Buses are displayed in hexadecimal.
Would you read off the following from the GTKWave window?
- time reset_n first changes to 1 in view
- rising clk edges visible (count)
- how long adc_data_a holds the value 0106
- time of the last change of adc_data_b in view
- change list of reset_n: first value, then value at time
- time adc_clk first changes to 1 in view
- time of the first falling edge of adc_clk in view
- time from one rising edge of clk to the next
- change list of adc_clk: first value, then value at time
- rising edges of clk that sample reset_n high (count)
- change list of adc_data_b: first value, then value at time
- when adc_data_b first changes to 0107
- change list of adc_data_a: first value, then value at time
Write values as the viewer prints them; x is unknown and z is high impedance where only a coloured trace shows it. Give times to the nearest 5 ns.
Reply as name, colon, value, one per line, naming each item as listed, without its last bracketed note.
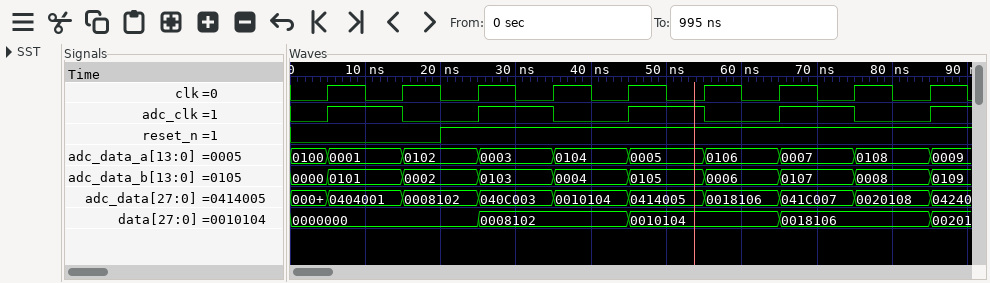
time reset_n first changes to 1 in view: 20 ns
rising clk edges visible: 9
how long adc_data_a holds the value 0106: 10 ns
time of the last change of adc_data_b in view: 85 ns
change list of reset_n: first value, then value at time: 0, 1 at 20 ns
time adc_clk first changes to 1 in view: 5 ns
time of the first falling edge of adc_clk in view: 15 ns
time from one rising edge of clk to the next: 10 ns
change list of adc_clk: first value, then value at time: 0, 1 at 5 ns, 0 at 15 ns, 1 at 25 ns, 0 at 35 ns, 1 at 45 ns, 0 at 55 ns, 1 at 65 ns, 0 at 75 ns, 1 at 85 ns
rising edges of clk that sample reset_n high: 7
change list of adc_data_b: first value, then value at time: 0000, 0101 at 5 ns, 0002 at 15 ns, 0103 at 25 ns, 0004 at 35 ns, 0105 at 45 ns, 0006 at 55 ns, 0107 at 65 ns, 0008 at 75 ns, 0109 at 85 ns
when adc_data_b first changes to 0107: 65 ns
change list of adc_data_a: first value, then value at time: 0100, 0001 at 5 ns, 0102 at 15 ns, 0003 at 25 ns, 0104 at 35 ns, 0005 at 45 ns, 0106 at 55 ns, 0007 at 65 ns, 0108 at 75 ns, 0009 at 85 ns
